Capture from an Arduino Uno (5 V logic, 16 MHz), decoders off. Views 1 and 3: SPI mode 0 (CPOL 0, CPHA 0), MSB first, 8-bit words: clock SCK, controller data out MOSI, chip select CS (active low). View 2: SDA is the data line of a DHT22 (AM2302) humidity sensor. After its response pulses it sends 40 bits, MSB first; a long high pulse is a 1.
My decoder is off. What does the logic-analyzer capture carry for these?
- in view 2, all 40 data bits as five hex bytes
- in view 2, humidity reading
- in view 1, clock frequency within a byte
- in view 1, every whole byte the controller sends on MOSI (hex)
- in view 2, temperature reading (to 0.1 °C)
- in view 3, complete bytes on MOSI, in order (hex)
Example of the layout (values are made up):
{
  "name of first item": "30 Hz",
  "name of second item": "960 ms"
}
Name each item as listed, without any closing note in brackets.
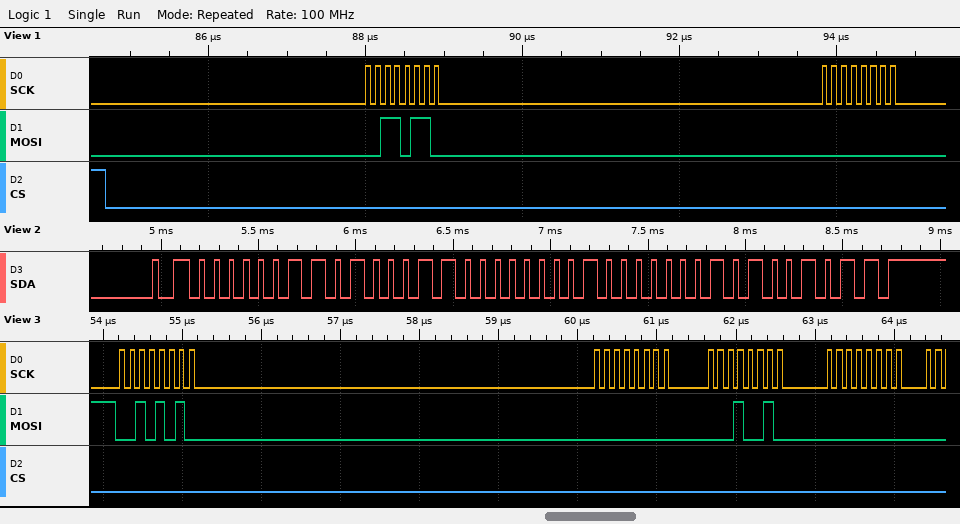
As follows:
{
  "in view 2, all 40 data bits as five hex bytes": "03 46 01 01 4B",
  "in view 2, humidity reading": "83.8 %",
  "in view 1, clock frequency within a byte": "8 MHz",
  "in view 1, every whole byte the controller sends on MOSI": "36 00",
  "in view 2, temperature reading": "25.7 °C",
  "in view 3, complete bytes on MOSI, in order": "0x2A 0x00 0x12 0x00"
}
